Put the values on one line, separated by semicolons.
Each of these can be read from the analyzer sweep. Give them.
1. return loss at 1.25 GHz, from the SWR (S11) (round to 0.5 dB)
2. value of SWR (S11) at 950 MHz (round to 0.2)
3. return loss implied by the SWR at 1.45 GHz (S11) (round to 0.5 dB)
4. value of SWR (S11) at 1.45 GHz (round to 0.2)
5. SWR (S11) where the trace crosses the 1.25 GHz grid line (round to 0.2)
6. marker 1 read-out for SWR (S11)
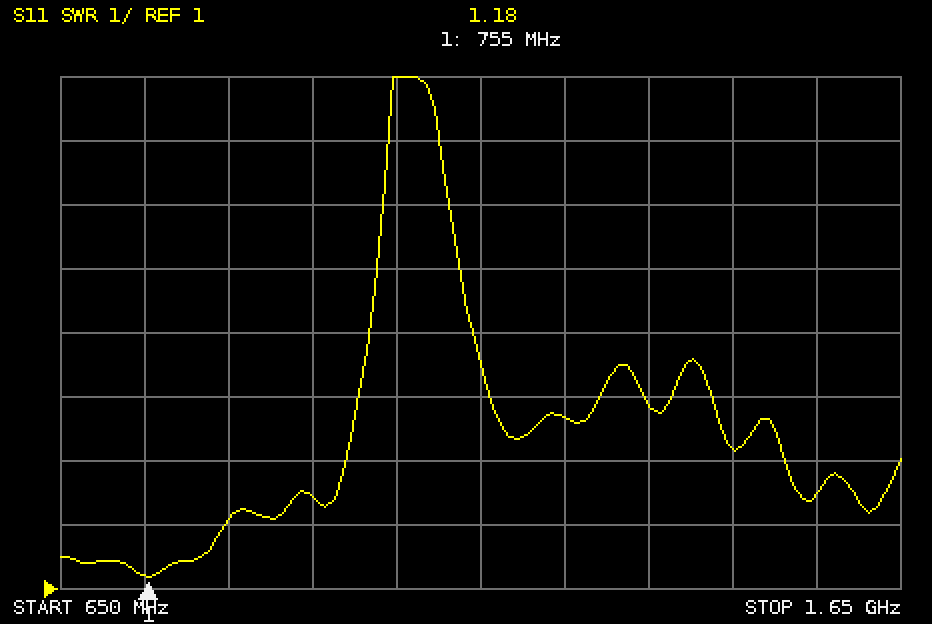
5.0 dB; 2.4; 5.5 dB; 3.2; 3.6; 1.18
